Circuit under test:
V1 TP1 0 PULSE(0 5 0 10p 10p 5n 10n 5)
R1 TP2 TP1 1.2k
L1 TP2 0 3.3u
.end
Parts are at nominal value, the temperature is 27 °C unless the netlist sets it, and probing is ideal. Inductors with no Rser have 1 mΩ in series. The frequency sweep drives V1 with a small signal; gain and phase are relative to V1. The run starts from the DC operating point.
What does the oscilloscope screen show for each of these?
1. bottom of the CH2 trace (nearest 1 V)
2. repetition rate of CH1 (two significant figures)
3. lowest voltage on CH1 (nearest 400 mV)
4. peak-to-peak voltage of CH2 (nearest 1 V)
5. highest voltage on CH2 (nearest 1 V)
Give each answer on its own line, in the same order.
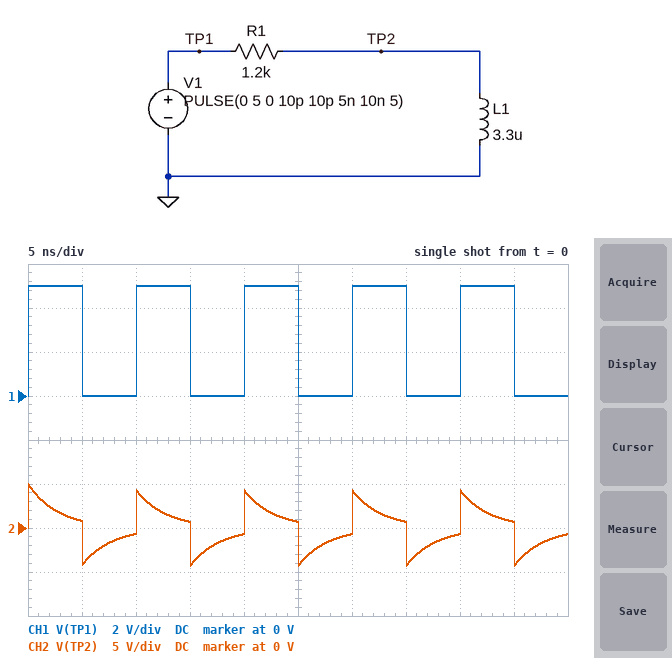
-4 V
100 MHz
0 V
9 V
5 V
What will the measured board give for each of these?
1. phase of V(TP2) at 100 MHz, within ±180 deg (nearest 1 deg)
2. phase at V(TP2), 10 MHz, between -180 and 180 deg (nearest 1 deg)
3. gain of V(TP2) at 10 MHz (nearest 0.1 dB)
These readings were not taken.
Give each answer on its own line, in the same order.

30 deg
80 deg
-15.4 dB
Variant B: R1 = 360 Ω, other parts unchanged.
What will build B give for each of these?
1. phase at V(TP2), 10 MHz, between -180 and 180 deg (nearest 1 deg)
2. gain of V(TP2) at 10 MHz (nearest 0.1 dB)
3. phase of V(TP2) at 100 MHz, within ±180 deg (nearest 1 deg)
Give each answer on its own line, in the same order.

60 deg
-6.0 dB
10 deg
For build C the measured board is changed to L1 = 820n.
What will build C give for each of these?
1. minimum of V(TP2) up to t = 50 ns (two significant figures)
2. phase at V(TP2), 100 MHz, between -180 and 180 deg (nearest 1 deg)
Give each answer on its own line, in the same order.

-5.0 V
67 deg
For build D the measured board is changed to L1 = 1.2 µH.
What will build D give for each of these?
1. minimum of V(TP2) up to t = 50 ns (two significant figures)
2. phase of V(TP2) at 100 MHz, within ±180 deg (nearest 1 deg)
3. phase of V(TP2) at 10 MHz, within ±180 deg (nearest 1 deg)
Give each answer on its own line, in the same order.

-4.9 V
58 deg
86 deg
